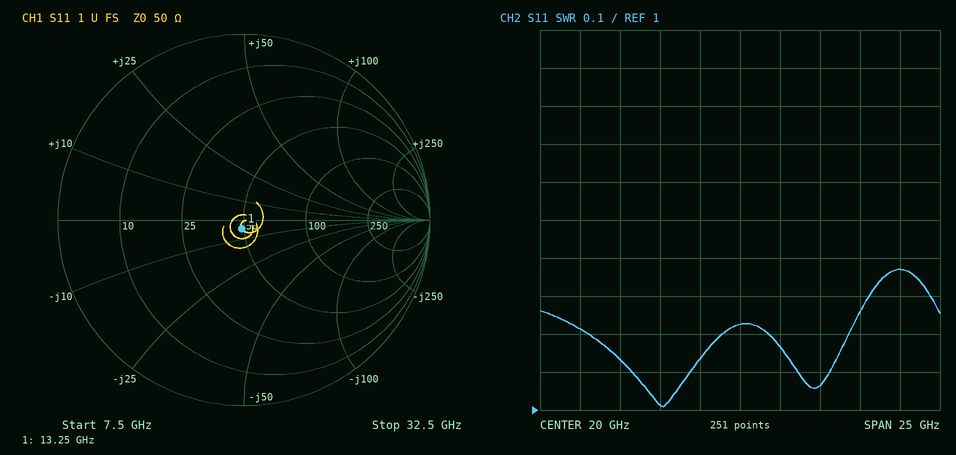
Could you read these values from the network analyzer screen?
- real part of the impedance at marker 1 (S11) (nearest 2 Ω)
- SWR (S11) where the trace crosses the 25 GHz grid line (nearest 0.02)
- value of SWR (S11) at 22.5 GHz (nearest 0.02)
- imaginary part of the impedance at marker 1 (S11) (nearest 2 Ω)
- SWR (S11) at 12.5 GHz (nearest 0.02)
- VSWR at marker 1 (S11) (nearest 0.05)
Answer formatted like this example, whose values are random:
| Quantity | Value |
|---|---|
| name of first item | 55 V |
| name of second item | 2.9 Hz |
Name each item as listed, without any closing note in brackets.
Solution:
| Quantity | Value |
|---|---|
| real part of the impedance at marker 1 (S11) | 48 Ω |
| SWR (S11) where the trace crosses the 25 GHz grid line | 1.06 |
| value of SWR (S11) at 22.5 GHz | 1.16 |
| imaginary part of the impedance at marker 1 (S11) | -4 Ω |
| SWR (S11) at 12.5 GHz | 1.14 |
| VSWR at marker 1 (S11) | 1.10 |
